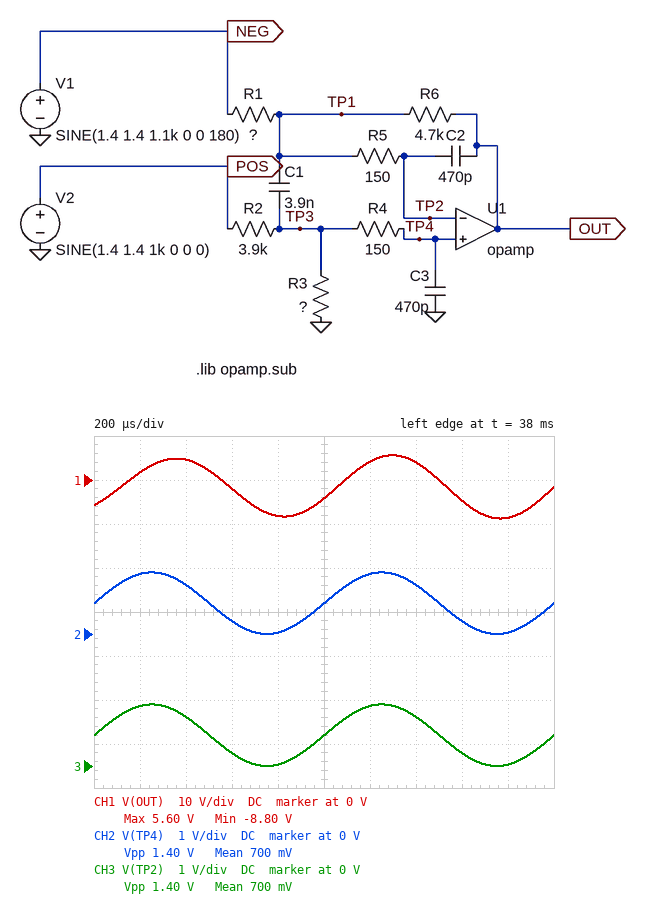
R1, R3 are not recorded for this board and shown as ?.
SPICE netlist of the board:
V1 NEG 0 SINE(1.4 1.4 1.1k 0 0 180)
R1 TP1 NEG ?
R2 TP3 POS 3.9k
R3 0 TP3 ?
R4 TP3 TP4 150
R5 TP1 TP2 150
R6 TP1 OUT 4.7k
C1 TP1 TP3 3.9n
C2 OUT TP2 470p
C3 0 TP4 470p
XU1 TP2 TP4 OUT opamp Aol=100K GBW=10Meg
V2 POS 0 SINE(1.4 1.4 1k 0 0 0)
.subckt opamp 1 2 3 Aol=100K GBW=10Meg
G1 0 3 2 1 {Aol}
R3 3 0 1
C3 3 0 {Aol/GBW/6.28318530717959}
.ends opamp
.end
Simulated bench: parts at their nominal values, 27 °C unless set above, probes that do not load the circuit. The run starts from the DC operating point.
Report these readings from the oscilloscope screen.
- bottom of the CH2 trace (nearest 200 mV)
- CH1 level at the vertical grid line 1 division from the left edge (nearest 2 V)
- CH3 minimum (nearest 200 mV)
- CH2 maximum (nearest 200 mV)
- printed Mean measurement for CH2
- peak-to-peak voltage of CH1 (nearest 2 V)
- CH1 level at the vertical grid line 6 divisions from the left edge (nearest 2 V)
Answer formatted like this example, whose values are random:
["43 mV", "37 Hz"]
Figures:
["0 V", "2 V", "0 V", "1.4 V", "700 mV", "14 V", "4 V"]
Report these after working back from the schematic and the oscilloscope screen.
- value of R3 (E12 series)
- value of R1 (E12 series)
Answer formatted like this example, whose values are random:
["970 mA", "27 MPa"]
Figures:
["3.9 kΩ", "1.5 kΩ"]
